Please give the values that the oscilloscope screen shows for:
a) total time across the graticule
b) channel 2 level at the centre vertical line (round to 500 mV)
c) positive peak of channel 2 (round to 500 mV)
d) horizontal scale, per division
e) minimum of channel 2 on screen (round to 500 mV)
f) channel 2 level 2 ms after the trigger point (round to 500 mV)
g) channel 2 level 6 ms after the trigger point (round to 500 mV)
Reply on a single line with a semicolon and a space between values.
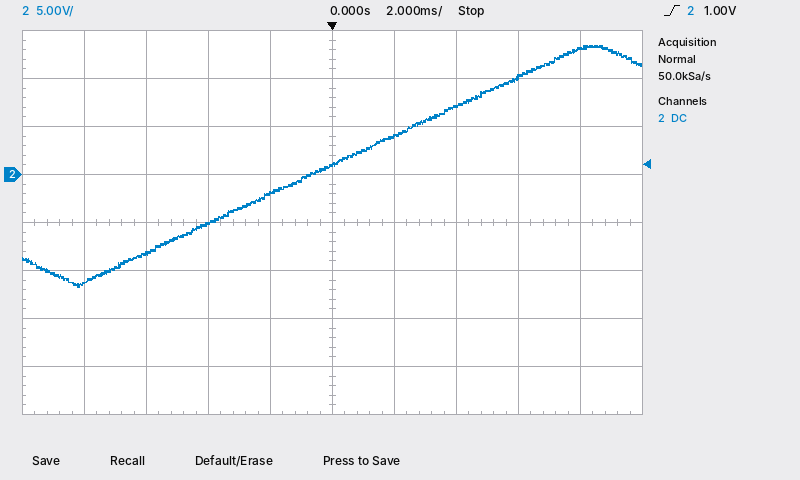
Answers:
20 ms; 1.0 V; 13.5 V; 2 ms; -12.0 V; 4.0 V; 10.0 V
